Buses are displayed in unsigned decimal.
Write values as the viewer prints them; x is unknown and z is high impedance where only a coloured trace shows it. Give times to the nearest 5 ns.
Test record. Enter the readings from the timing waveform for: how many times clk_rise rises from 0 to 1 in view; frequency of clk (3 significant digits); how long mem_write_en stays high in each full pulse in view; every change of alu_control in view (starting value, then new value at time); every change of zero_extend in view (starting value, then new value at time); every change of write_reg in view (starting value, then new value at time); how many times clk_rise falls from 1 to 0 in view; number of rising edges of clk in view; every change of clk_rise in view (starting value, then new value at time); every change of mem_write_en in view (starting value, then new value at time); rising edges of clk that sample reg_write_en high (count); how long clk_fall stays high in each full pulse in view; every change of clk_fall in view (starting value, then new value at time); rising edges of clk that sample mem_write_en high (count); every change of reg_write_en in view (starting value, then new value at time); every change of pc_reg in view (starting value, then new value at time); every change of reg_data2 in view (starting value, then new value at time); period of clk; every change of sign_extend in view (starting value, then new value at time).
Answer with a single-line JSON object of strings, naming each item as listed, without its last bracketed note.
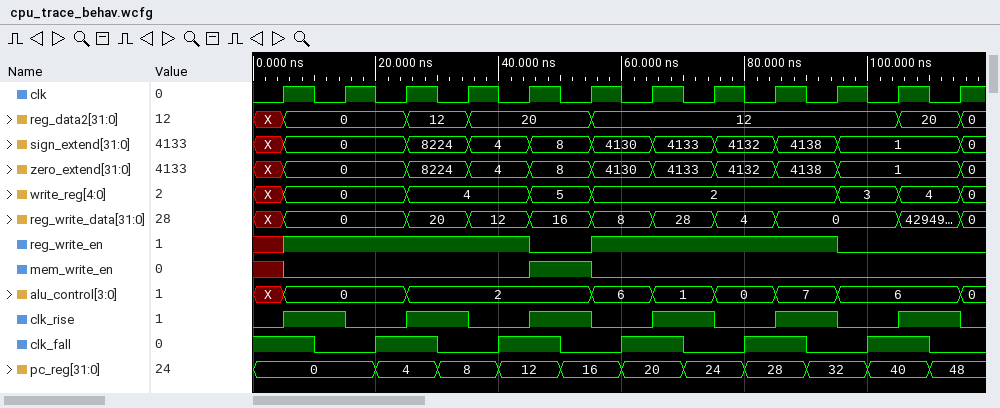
{"how many times clk_rise rises from 0 to 1 in view": "6", "frequency of clk": "100 MHz", "how long mem_write_en stays high in each full pulse in view": "10 ns", "every change of alu_control in view": "X, 0 at 5 ns, 2 at 25 ns, 6 at 55 ns, 1 at 65 ns, 0 at 75 ns, 7 at 85 ns, 6 at 95 ns, 0 at 115 ns", "every change of zero_extend in view": "X, 0 at 5 ns, 8224 at 25 ns, 4 at 35 ns, 8 at 45 ns, 4130 at 55 ns, 4133 at 65 ns, 4132 at 75 ns, 4138 at 85 ns, 1 at 95 ns, 0 at 115 ns", "every change of write_reg in view": "X, 0 at 5 ns, 4 at 25 ns, 5 at 45 ns, 2 at 55 ns, 3 at 95 ns, 4 at 105 ns, 0 at 115 ns", "how many times clk_rise falls from 1 to 0 in view": "6", "number of rising edges of clk in view": "12", "every change of clk_rise in view": "0, 1 at 5 ns, 0 at 15 ns, 1 at 25 ns, 0 at 35 ns, 1 at 45 ns, 0 at 55 ns, 1 at 65 ns, 0 at 75 ns, 1 at 85 ns, 0 at 95 ns, 1 at 105 ns, 0 at 115 ns", "every change of mem_write_en in view": "x, 0 at 5 ns, 1 at 45 ns, 0 at 55 ns", "rising edges of clk that sample reg_write_en high": "8", "how long clk_fall stays high in each full pulse in view": "10 ns, 10 ns, 10 ns, 10 ns, 10 ns", "every change of clk_fall in view": "1, 0 at 10 ns, 1 at 20 ns, 0 at 30 ns, 1 at 40 ns, 0 at 50 ns, 1 at 60 ns, 0 at 70 ns, 1 at 80 ns, 0 at 90 ns, 1 at 100 ns, 0 at 110 ns", "rising edges of clk that sample mem_write_en high": "1", "every change of reg_write_en in view": "x, 1 at 5 ns, 0 at 45 ns, 1 at 55 ns, 0 at 95 ns", "every change of pc_reg in view": "0, 4 at 20 ns, 8 at 30 ns, 12 at 40 ns, 16 at 50 ns, 20 at 60 ns, 24 at 70 ns, 28 at 80 ns, 32 at 90 ns, 40 at 100 ns, 48 at 110 ns", "every change of reg_data2 in view": "X, 0 at 5 ns, 12 at 25 ns, 20 at 35 ns, 12 at 55 ns, 20 at 105 ns, 0 at 115 ns", "period of clk": "10 ns", "every change of sign_extend in view": "X, 0 at 5 ns, 8224 at 25 ns, 4 at 35 ns, 8 at 45 ns, 4130 at 55 ns, 4133 at 65 ns, 4132 at 75 ns, 4138 at 85 ns, 1 at 95 ns, 0 at 115 ns"}
